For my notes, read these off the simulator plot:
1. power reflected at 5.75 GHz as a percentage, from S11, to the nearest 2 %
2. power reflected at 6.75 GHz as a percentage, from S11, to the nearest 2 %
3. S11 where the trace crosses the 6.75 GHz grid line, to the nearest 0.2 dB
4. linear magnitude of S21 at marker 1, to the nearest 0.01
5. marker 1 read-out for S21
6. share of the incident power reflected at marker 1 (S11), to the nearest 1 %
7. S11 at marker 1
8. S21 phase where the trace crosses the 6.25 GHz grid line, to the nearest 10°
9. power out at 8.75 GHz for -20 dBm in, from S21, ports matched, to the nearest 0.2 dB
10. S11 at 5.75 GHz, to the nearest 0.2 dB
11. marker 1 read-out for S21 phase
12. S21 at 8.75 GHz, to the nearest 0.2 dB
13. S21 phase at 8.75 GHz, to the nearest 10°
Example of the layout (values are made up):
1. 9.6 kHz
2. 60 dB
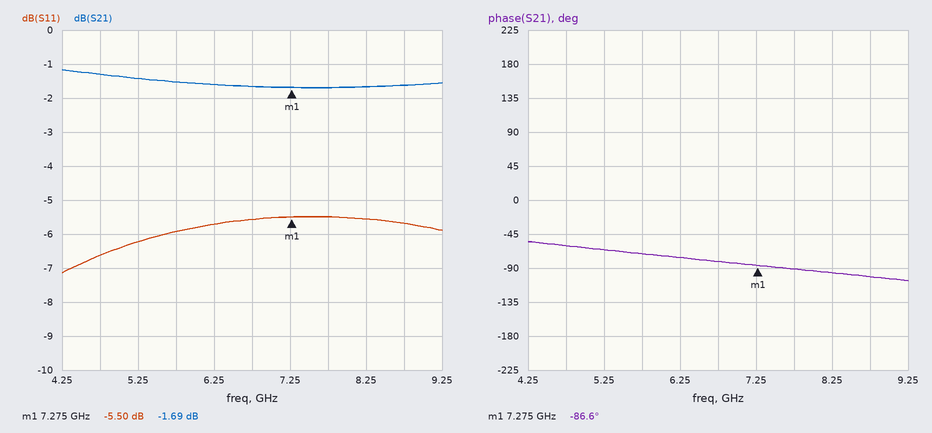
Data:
1. 26 %
2. 28 %
3. -5.6 dB
4. 0.82
5. -1.69 dB
6. 28 %
7. -5.50 dB
8. -80°
9. -21.6 dBm
10. -6.0 dB
11. -86.6°
12. -1.6 dB
13. -100°
